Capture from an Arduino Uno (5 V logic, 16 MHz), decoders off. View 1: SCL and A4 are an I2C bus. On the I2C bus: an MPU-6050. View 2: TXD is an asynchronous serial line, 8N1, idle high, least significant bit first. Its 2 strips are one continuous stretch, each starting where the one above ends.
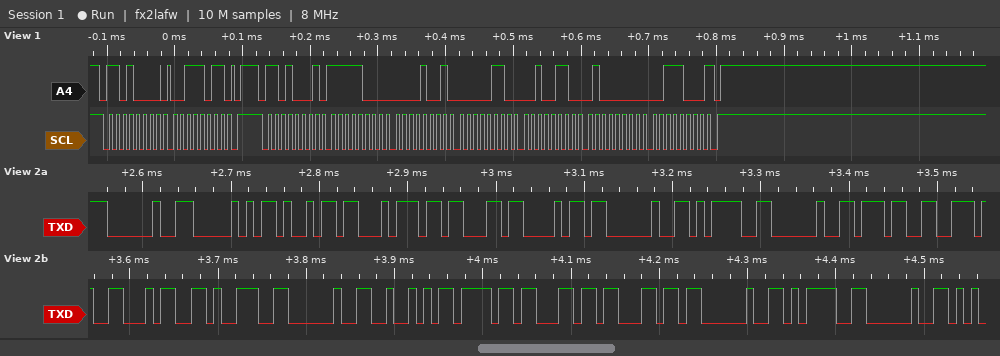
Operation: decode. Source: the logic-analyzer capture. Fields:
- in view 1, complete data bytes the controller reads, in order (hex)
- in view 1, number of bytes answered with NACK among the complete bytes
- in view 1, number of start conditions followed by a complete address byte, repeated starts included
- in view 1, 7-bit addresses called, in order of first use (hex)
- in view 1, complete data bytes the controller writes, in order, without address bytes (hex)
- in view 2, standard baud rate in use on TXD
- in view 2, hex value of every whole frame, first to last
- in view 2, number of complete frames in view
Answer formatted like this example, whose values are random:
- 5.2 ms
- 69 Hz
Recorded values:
- F8 09 06 26 40 38
- 1
- 2
- 0x68
- 3B
- 115200 baud
- 20 50 69 74 63 68 20 3D 20 37 2E 34 39 20 52 6F 6C 6C 20 3D 20
- 21
